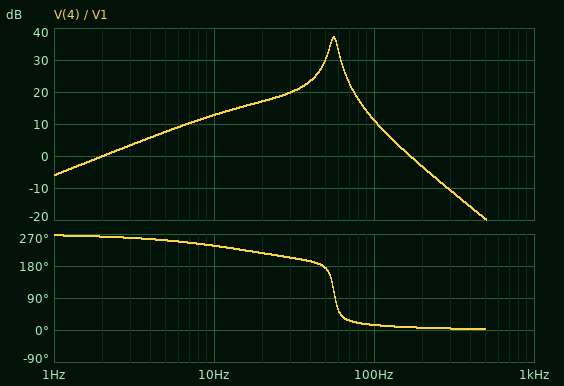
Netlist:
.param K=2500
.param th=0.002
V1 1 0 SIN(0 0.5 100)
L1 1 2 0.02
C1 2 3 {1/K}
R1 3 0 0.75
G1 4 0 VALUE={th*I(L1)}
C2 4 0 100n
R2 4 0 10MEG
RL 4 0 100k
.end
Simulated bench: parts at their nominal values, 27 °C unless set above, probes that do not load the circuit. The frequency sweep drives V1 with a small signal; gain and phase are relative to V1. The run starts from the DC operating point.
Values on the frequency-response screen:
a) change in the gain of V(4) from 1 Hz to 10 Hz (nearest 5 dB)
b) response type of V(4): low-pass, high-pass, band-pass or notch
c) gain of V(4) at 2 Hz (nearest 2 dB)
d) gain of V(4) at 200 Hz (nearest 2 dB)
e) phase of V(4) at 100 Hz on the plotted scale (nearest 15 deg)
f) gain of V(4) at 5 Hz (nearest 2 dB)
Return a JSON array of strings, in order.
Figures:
["20 dB", "band-pass", "0 dB", "-4 dB", "15 deg", "8 dB"]
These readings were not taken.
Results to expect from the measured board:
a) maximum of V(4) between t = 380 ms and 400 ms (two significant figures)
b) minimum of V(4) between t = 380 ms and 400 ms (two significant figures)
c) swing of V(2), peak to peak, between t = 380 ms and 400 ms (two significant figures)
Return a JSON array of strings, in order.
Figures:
["1.8 V", "-1.8 V", "470 mV"]
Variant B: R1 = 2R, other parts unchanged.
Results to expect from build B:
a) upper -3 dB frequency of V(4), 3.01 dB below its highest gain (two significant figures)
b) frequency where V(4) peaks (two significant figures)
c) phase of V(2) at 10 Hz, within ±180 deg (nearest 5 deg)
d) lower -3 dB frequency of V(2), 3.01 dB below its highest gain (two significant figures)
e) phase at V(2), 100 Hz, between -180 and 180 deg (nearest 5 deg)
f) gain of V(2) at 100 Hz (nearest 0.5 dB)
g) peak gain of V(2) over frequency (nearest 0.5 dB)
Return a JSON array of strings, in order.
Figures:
["63 Hz", "55 Hz", "0 deg", "47 Hz", "-140 deg", "-6.0 dB", "11.5 dB"]
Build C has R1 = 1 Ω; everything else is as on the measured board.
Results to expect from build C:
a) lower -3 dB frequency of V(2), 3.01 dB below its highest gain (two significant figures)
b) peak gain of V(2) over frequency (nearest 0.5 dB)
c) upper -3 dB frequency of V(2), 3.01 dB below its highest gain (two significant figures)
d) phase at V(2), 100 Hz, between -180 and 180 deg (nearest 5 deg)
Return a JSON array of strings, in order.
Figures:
["52 Hz", "17.0 dB", "60 Hz", "-160 deg"]
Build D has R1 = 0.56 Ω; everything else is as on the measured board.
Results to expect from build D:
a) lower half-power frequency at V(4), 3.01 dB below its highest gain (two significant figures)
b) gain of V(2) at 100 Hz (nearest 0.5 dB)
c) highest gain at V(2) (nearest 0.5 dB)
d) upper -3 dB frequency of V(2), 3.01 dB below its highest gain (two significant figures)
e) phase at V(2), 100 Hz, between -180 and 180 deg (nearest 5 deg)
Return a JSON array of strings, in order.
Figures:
["54 Hz", "-6.5 dB", "22.0 dB", "58 Hz", "-170 deg"]
